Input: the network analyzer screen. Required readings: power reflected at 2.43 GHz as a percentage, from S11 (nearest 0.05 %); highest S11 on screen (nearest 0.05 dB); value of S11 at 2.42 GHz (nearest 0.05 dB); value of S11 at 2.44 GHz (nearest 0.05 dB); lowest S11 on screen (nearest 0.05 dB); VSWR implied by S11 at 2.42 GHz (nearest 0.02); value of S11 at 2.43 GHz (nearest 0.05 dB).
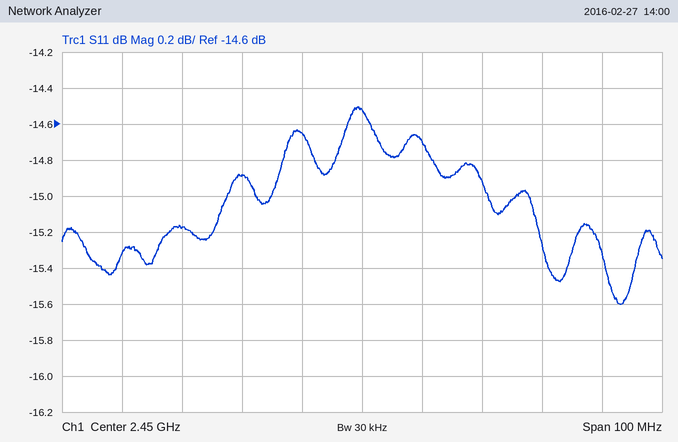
3.25 %
-14.50 dB
-15.15 dB
-14.65 dB
-15.60 dB
1.42
-14.90 dB
